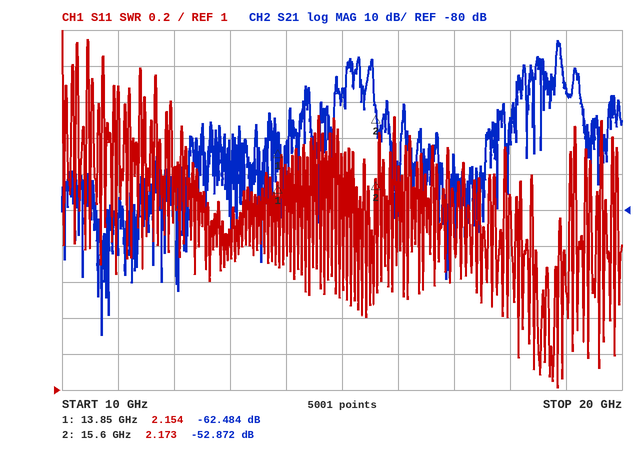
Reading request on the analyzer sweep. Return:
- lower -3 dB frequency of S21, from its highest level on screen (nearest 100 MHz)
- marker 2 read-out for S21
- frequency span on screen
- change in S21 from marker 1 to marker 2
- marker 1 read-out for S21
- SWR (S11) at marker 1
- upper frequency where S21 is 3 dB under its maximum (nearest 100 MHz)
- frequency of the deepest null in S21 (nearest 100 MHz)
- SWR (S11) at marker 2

18.8 GHz
-52.872 dB
10 GHz
9.612 dB
-62.484 dB
2.154
18.9 GHz
10.7 GHz
2.173
